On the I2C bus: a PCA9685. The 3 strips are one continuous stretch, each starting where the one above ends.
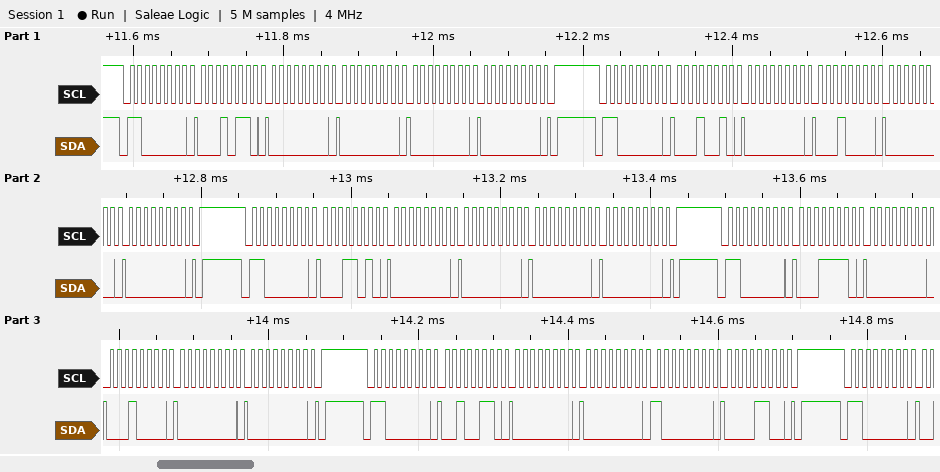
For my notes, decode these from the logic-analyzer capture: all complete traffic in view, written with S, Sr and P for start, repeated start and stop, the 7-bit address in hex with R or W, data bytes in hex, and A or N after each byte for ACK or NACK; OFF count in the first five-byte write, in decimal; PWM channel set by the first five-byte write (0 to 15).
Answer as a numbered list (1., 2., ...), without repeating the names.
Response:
1. S 60W A 16 A 00 A 00 A 00 A 00 A P S 60W A 12 A 00 A 10 A 00 A 00 A P S 60W A 1A A 00 A 00 A 00 A 00 A P S 60W A 1E A 00 A 10 A 00 A 00 A P S 60W A 26 A 00 A 00 A 80 A 0C A P S 60W A
2. 0
3. 4
